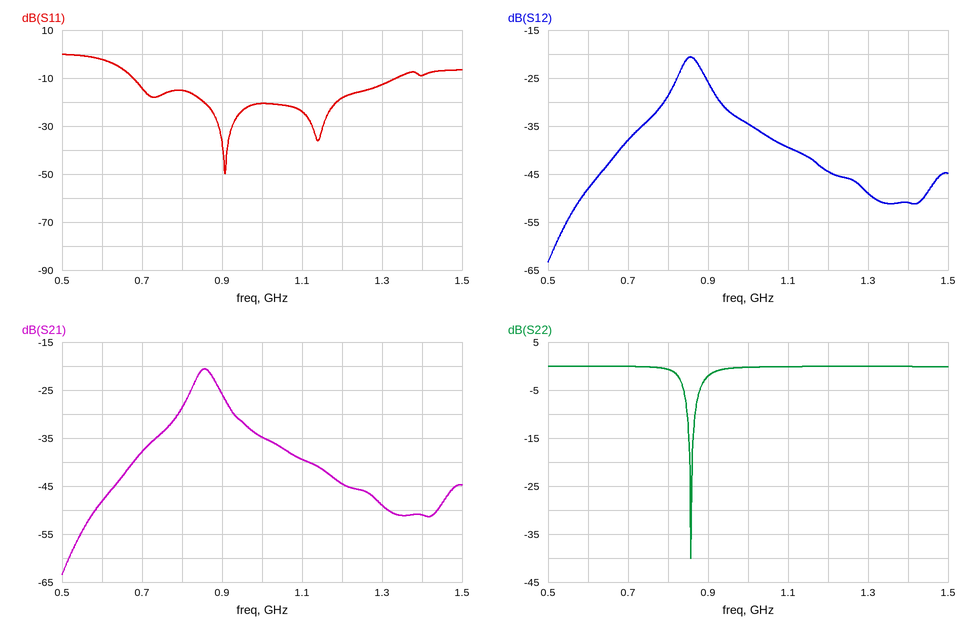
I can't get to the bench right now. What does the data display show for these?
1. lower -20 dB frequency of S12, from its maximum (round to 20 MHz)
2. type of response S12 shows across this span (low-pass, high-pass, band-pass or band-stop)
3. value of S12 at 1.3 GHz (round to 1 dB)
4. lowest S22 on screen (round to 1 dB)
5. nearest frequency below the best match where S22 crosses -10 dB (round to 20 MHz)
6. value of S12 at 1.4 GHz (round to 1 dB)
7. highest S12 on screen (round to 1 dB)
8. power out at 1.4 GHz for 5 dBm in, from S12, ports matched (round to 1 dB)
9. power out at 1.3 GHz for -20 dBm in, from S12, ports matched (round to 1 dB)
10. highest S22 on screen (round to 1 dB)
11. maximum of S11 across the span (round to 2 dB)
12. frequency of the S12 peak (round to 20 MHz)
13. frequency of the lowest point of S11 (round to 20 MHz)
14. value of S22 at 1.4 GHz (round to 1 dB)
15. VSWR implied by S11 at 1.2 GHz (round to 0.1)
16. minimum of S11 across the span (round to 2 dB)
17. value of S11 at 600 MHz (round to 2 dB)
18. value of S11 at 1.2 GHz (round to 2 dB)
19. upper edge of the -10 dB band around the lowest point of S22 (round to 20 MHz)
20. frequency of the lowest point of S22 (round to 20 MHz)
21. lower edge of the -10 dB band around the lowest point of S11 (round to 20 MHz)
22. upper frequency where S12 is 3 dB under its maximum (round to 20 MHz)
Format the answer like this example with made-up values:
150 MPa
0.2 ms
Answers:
680 MHz
band-pass
-49 dB
-40 dB
840 MHz
-51 dB
-21 dB
-46 dBm
-69 dBm
0 dB
0 dB
860 MHz
900 MHz
0 dB
1.3
-50 dB
-2 dB
-18 dB
860 MHz
860 MHz
680 MHz
880 MHz
